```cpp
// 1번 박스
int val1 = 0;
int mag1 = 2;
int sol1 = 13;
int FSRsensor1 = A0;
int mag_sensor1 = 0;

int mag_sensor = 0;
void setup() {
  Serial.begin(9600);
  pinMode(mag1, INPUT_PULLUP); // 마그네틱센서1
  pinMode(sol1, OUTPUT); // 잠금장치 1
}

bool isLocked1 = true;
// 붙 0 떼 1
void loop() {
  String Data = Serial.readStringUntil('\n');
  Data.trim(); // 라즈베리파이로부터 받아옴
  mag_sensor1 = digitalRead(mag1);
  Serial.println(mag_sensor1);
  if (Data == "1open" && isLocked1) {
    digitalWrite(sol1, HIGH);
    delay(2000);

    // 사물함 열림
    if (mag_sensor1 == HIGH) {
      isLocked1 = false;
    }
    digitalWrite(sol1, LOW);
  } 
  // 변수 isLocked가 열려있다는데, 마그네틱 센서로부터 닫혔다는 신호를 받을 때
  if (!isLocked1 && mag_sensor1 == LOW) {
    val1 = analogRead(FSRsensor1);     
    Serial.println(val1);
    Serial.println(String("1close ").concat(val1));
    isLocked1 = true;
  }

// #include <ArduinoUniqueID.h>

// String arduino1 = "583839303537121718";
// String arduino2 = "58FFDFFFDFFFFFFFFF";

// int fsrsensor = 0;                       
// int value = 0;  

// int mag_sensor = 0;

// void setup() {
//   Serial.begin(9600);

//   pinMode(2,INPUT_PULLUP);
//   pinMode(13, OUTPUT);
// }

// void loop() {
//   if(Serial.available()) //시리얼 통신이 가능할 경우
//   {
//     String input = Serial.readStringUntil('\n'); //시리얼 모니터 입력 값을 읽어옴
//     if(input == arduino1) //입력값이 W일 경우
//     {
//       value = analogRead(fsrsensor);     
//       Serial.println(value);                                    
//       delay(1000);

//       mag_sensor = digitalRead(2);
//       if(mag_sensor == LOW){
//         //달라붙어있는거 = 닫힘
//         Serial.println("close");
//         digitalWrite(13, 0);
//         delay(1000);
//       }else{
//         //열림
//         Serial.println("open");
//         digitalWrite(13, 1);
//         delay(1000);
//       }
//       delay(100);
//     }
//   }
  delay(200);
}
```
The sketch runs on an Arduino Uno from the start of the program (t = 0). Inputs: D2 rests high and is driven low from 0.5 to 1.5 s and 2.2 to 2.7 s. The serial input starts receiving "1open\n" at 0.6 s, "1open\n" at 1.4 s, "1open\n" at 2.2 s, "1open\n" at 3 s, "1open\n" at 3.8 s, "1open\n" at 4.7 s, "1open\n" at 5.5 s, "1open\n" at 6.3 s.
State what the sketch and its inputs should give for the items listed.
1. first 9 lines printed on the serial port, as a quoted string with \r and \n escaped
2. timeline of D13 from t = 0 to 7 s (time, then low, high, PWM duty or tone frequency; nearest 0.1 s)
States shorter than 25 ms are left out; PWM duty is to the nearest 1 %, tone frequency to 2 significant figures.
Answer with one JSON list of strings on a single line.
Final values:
["\"0\\r\\n1\\r\\n1\\r\\n1\\r\\n1\\r\\n1\\r\\n1\\r\\n1\\r\\n1\\r\\n\"", "0 s low; 0.6 s high; 2.6 s low; 2.8 s high; 4.8 s low"]
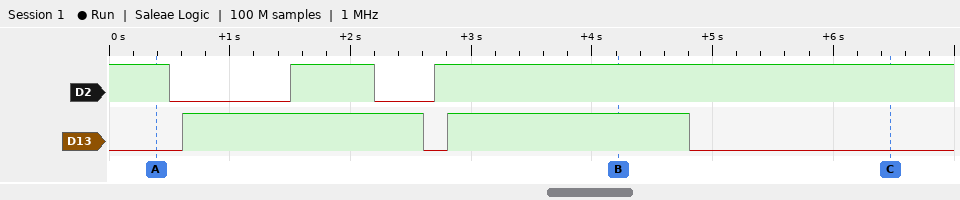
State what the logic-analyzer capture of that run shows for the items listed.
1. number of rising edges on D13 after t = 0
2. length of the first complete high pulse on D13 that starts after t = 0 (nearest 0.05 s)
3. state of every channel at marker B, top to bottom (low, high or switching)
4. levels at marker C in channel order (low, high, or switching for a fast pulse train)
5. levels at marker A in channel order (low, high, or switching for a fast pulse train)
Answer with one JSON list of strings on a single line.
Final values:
["2", "2.00 s", "D2 high, D13 high", "D2 high, D13 low", "D2 high, D13 low"]
